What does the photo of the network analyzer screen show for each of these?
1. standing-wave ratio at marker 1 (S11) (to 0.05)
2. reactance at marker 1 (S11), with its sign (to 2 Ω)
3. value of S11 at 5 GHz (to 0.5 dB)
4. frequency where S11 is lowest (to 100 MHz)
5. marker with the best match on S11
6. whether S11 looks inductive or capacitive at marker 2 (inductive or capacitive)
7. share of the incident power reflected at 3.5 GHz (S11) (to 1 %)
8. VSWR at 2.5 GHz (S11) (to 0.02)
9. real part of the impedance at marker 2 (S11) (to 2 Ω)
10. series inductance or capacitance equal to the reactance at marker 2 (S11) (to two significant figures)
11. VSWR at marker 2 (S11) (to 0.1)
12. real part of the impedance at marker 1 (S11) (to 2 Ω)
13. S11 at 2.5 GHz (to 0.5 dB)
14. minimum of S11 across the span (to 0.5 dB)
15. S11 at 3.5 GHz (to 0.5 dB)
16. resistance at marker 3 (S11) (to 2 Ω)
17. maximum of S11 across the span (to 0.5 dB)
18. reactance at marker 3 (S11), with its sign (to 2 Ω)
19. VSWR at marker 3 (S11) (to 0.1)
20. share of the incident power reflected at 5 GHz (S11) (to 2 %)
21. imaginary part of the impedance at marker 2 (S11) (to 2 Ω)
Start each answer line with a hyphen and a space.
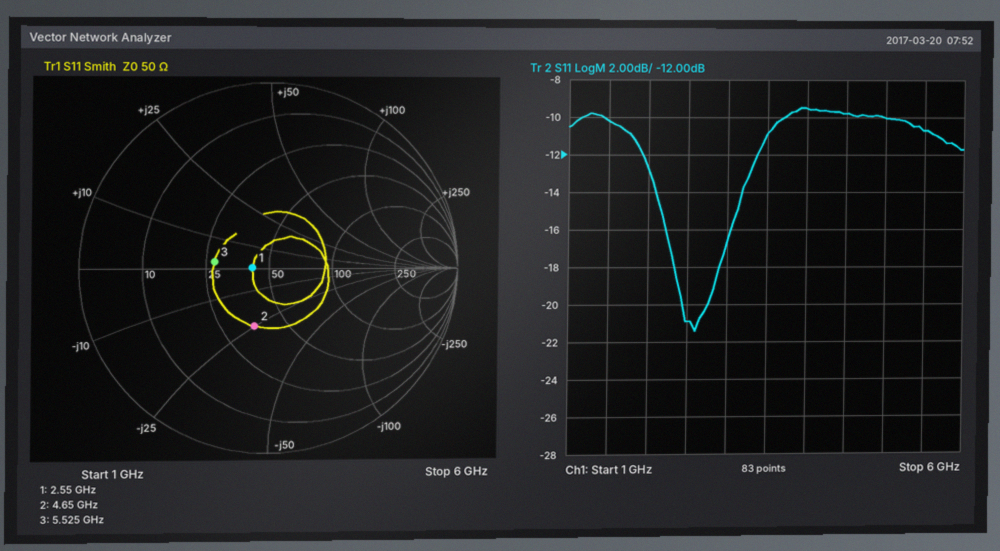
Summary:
- 1.20
- 0 Ω
- -10.0 dB
- 2.6 GHz
- marker 1
- capacitive
- 8 %
- 1.20
- 36 Ω
- 1.4 pF
- 1.9
- 42 Ω
- -21.0 dB
- -21.5 dB
- -11.0 dB
- 28 Ω
- -9.5 dB
- +2 Ω
- 1.8
- 10 %
- -24 Ω
